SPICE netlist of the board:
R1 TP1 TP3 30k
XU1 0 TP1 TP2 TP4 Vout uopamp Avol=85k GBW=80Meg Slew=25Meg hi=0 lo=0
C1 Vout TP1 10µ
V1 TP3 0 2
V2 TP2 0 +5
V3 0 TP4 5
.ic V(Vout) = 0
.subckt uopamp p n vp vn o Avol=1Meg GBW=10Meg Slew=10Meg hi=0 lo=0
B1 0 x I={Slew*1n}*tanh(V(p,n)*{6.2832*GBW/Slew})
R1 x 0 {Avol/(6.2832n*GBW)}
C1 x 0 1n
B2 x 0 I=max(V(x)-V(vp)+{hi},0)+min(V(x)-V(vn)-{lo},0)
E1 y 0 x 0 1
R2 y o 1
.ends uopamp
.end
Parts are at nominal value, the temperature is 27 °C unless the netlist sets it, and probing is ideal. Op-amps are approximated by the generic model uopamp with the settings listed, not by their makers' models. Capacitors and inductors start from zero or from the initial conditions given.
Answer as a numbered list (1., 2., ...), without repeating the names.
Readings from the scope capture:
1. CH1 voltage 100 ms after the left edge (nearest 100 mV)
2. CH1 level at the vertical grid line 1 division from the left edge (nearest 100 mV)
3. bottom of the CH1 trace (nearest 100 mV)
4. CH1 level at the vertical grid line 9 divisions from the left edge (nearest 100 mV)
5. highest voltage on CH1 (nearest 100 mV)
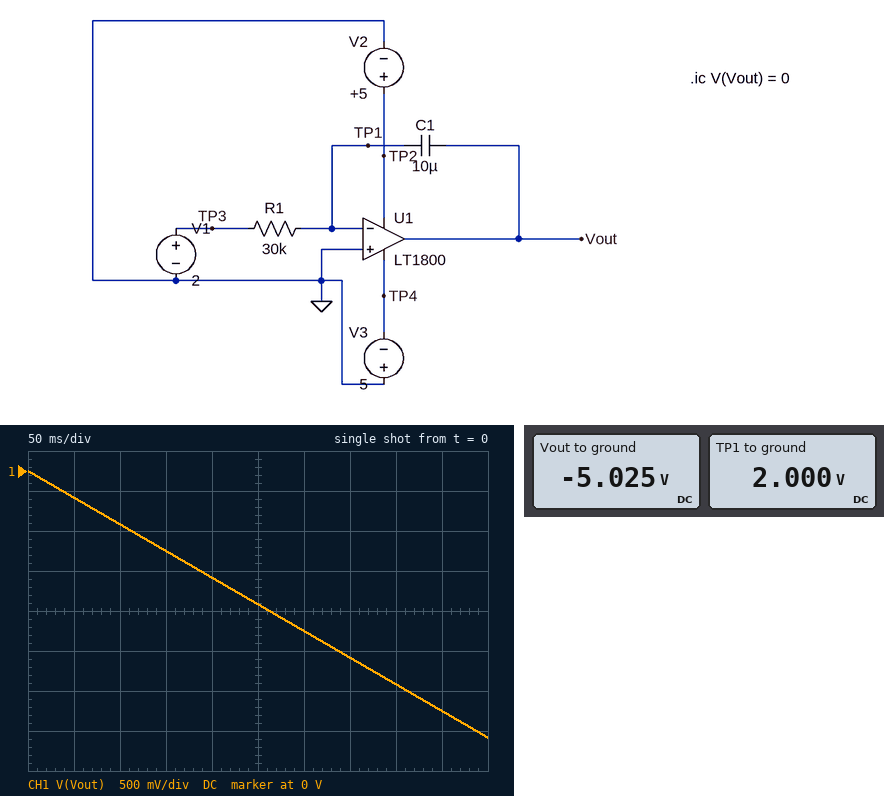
1. -700 mV
2. -300 mV
3. -3.3 V
4. -3.0 V
5. 0 V
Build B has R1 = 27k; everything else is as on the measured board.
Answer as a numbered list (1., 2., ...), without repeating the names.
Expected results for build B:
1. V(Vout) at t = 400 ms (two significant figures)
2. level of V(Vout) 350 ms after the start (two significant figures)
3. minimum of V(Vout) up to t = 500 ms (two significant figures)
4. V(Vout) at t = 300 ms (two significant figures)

1. -3.0 V
2. -2.6 V
3. -3.7 V
4. -2.2 V
